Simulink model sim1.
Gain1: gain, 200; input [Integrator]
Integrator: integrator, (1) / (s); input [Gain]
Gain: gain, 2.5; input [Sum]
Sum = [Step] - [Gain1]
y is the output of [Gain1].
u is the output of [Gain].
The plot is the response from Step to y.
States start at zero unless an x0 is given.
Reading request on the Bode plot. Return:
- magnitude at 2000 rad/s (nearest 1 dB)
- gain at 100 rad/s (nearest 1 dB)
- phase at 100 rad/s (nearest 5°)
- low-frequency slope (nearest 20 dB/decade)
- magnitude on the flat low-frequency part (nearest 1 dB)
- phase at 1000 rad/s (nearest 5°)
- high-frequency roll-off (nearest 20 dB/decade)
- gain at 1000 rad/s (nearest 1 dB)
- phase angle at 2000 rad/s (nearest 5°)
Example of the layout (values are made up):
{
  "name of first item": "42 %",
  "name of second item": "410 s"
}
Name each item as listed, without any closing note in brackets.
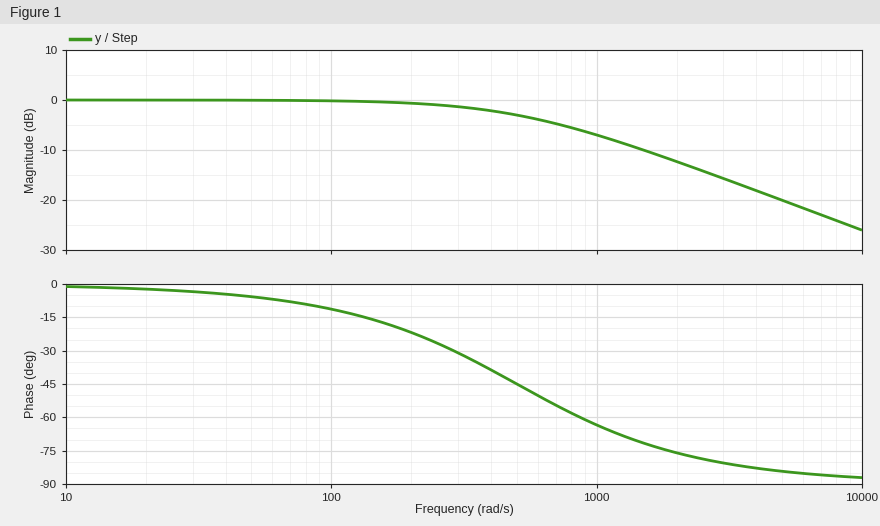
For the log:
{
  "magnitude at 2000 rad/s": "-12 dB",
  "gain at 100 rad/s": "0 dB",
  "phase at 100 rad/s": "-10°",
  "low-frequency slope": "0 dB/decade",
  "magnitude on the flat low-frequency part": "0 dB",
  "phase at 1000 rad/s": "-65°",
  "high-frequency roll-off": "-20 dB/decade",
  "gain at 1000 rad/s": "-7 dB",
  "phase angle at 2000 rad/s": "-75°"
}
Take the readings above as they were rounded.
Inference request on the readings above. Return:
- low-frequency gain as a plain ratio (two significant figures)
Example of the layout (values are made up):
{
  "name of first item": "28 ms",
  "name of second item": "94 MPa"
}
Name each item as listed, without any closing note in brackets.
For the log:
{
  "low-frequency gain as a plain ratio": "1.0"
}
